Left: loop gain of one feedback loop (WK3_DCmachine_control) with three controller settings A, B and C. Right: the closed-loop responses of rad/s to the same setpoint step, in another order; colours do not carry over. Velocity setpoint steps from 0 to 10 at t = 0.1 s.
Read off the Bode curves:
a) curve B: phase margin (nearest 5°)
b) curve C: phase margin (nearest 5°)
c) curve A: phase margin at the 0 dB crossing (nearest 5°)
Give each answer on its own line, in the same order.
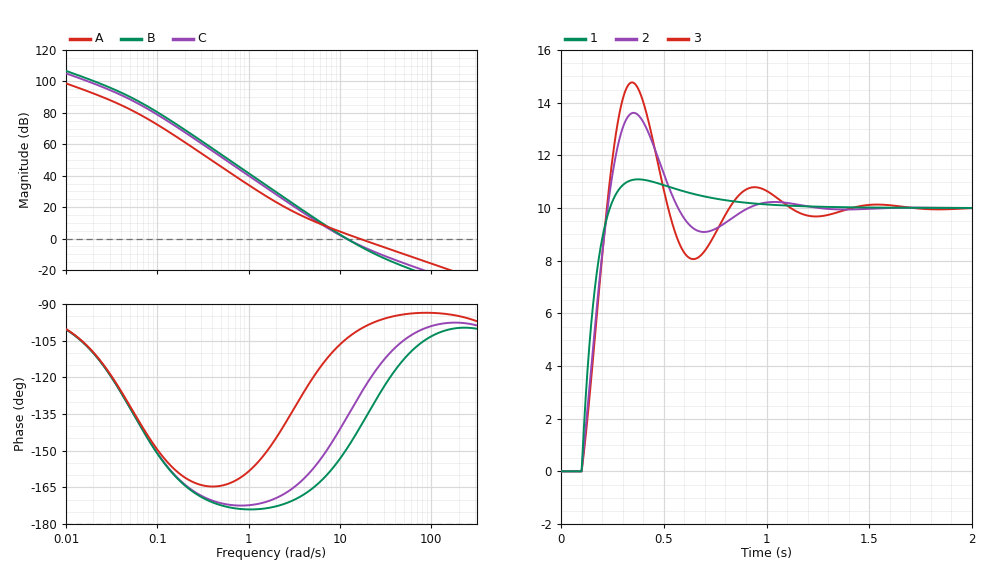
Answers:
30°
45°
80°
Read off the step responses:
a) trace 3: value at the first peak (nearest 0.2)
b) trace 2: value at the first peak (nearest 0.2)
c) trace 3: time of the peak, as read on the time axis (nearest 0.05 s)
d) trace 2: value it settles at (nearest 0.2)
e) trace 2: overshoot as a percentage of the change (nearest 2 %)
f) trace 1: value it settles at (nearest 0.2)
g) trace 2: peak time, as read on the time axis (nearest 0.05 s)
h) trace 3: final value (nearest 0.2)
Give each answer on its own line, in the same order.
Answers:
14.8
13.6
0.35 s
10.0
36 %
10.0
0.35 s
10.0
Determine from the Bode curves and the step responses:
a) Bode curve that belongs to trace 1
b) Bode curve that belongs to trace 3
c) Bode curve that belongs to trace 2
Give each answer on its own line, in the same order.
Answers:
A
B
C
